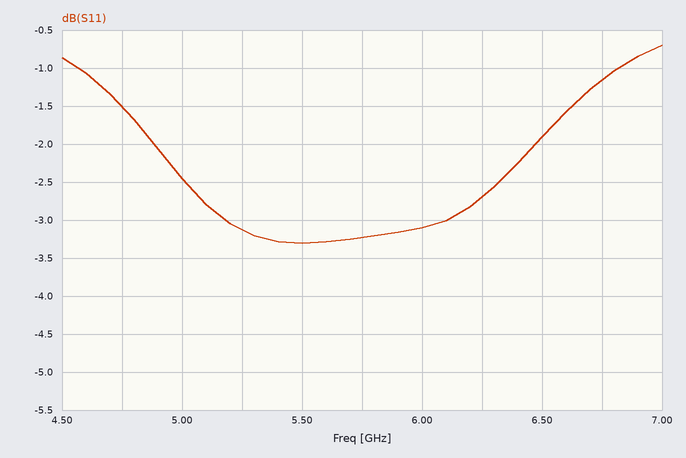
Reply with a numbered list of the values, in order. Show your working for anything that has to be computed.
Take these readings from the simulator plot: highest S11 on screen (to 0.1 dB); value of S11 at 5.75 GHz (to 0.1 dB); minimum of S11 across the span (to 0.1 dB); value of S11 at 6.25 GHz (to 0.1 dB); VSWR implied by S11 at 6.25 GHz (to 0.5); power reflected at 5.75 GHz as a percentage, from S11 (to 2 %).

1. -0.7 dB
2. -3.2 dB
3. -3.3 dB
4. -2.7 dB
5. |Γ| = 10^(-2.7/20) = 0.7328; VSWR = (1 + 0.7328)/(1 − 0.7328) ≈ 6.5
6. 10^(-3.2/10) ≈ 48 %
